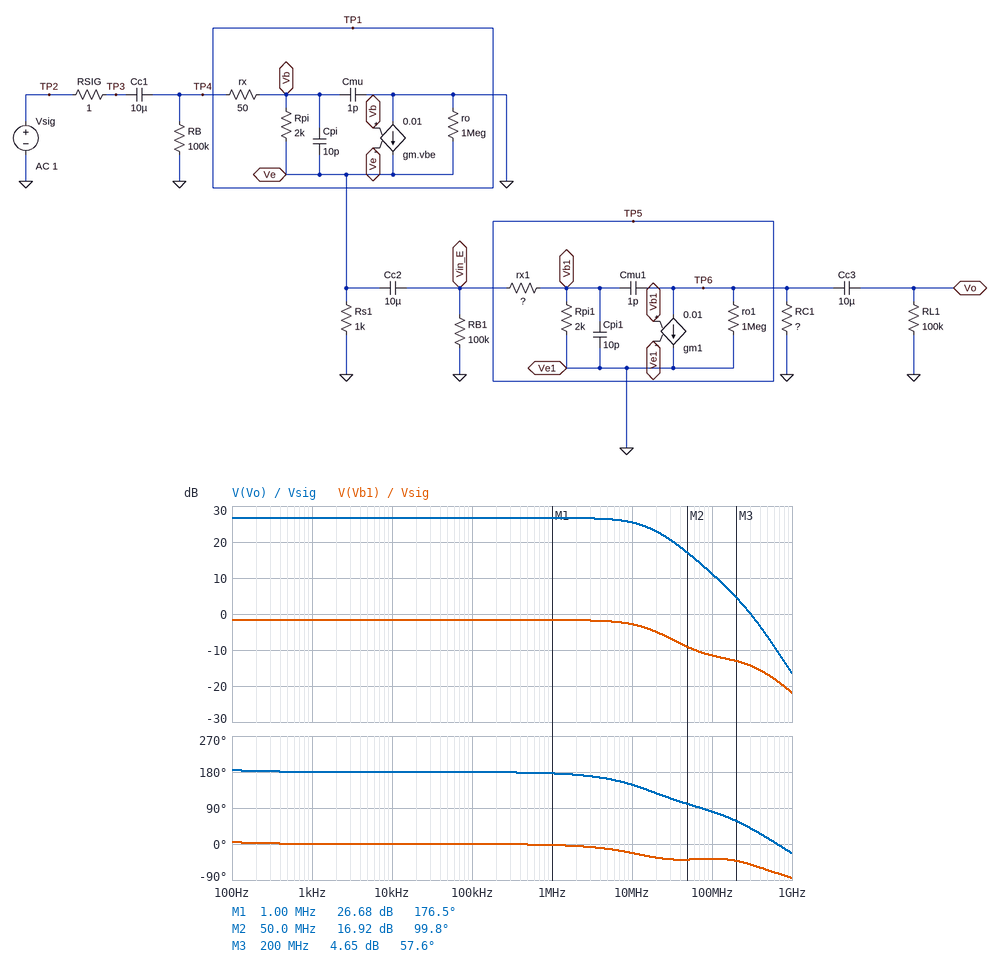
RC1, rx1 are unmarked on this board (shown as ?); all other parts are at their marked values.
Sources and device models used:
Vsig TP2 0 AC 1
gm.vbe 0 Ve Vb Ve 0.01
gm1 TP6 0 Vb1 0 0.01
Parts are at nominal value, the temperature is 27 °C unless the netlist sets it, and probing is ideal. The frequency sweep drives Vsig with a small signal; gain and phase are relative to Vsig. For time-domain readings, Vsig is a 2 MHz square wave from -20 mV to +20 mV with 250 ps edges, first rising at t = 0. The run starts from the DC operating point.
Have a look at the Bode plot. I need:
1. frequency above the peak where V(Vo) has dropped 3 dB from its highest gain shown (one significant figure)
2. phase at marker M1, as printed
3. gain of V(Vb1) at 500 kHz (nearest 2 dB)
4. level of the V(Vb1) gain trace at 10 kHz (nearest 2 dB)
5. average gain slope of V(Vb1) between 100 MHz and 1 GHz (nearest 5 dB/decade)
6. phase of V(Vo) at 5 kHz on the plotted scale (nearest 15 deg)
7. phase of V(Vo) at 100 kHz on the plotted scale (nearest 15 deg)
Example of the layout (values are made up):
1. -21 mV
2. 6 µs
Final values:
1. 20 MHz
2. 176.5 deg
3. -2 dB
4. -2 dB
5. -10 dB/decade
6. 180 deg
7. 180 deg
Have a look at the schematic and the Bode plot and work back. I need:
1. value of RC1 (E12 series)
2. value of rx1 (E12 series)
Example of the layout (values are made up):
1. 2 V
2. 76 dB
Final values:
1. 2.7 kΩ
2. 120 Ω
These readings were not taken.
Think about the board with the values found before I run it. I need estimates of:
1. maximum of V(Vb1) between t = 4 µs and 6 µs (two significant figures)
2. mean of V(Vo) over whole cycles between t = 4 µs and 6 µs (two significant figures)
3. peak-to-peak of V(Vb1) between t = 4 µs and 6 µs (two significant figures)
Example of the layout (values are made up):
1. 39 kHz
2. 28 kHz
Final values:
1. 33 mV
2. -430 mV
3. 33 mV
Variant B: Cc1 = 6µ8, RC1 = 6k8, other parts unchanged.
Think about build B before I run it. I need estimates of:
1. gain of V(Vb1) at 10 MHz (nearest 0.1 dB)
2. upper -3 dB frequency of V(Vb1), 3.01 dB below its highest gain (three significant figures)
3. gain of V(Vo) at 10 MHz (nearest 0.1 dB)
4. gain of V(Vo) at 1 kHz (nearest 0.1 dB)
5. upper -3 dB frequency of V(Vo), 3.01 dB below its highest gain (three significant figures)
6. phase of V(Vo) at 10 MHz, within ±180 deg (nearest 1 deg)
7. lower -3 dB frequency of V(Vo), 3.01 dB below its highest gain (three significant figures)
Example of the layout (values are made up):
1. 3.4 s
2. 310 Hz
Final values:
1. -5.1 dB
2. 8.96 MHz
3. 30.3 dB
4. 34.3 dB
5. 8.00 MHz
6. 127 deg
7. 8.03 Hz
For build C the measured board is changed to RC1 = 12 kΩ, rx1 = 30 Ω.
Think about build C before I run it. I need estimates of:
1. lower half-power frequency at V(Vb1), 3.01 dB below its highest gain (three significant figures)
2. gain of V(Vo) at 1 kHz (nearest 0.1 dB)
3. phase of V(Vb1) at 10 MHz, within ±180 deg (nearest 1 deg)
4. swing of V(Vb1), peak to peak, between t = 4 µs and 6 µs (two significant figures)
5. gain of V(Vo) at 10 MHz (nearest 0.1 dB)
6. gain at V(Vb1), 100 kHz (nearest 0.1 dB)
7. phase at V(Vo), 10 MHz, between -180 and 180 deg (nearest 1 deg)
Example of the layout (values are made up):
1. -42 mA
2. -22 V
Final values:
1. 8.08 Hz
2. 39.2 dB
3. -23 deg
4. 34 mV
5. 34.2 dB
6. -1.3 dB
7. 123 deg
